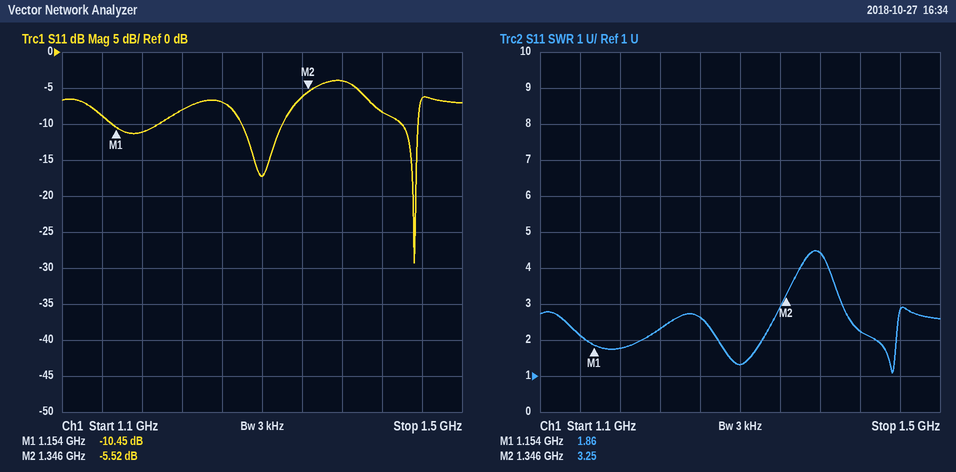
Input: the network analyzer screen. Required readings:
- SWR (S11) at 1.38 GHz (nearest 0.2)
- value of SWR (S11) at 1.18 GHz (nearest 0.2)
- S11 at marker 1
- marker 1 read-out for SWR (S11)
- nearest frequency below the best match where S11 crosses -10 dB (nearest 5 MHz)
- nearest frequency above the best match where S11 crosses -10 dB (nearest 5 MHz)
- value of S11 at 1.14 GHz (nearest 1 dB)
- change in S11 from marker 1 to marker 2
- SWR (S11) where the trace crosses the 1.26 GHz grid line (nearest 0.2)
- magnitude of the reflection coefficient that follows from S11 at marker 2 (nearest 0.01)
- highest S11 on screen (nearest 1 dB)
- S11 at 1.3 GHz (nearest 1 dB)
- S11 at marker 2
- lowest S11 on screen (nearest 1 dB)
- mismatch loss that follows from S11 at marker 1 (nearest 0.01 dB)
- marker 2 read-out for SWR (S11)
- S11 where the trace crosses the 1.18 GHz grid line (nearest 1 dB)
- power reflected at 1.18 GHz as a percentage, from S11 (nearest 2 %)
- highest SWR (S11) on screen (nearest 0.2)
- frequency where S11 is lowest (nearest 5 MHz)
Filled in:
4.4
1.8
-10.45 dB
1.86
1.440 GHz
1.455 GHz
-9 dB
4.93 dB
2.6
0.53
-4 dB
-17 dB
-5.52 dB
-29 dB
0.41 dB
3.25
-11 dB
8 %
4.4
1.450 GHz
